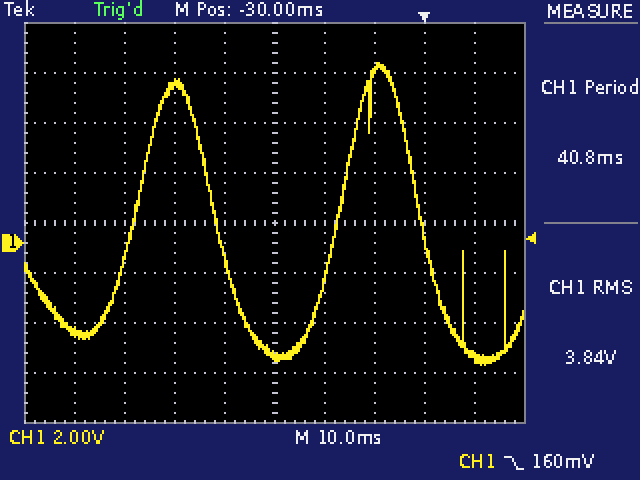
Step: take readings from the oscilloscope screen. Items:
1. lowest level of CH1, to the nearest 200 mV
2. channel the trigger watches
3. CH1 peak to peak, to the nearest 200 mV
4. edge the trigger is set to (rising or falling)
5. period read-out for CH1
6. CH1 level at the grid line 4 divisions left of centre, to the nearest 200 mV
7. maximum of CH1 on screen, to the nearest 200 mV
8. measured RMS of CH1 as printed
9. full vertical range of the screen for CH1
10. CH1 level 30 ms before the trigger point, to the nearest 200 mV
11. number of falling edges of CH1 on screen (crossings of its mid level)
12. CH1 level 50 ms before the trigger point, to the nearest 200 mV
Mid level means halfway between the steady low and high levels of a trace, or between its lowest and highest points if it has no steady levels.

-4.8 V
CH1
12.0 V
falling
40.8 ms
-3.6 V
7.2 V
3.84 V
16 V
-4.6 V
2
6.4 V
